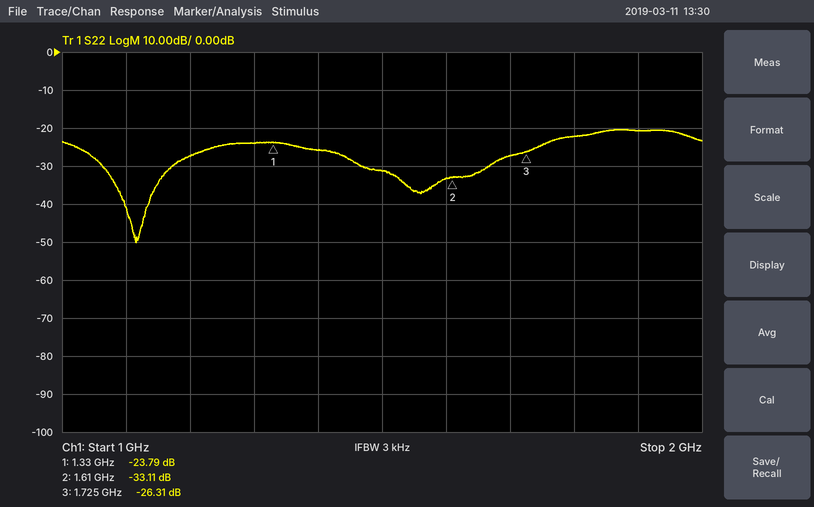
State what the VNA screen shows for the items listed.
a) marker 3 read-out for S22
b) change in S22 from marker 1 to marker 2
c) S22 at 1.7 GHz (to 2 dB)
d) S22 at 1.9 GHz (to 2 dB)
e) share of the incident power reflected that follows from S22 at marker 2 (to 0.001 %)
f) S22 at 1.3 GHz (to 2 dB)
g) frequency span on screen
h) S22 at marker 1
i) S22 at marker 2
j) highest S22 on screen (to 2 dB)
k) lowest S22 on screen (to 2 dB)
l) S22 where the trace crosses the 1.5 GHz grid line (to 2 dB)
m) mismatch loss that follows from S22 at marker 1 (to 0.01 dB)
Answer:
-26.31 dB
-9.32 dB
-28 dB
-20 dB
0.049 %
-24 dB
1 GHz
-23.79 dB
-33.11 dB
-20 dB
-50 dB
-32 dB
0.02 dB
